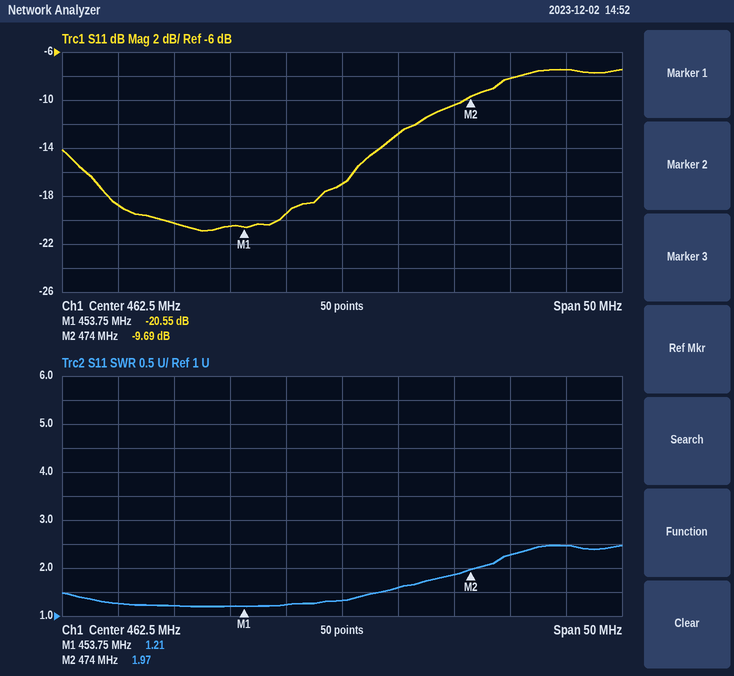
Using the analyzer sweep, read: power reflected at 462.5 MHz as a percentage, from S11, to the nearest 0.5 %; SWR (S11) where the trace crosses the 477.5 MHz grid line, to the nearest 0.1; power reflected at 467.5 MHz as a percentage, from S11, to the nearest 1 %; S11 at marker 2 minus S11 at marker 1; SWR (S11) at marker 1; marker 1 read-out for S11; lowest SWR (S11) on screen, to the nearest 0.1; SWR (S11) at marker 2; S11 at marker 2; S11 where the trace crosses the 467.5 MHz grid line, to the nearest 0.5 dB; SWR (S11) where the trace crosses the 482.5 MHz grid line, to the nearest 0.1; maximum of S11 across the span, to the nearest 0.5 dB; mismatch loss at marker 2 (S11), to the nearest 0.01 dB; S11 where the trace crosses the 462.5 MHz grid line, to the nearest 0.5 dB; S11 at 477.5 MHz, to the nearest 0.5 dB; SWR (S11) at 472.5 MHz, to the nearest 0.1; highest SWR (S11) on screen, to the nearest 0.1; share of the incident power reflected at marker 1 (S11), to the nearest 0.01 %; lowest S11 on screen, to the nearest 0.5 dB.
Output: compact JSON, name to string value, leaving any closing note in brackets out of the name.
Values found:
{"power reflected at 462.5 MHz as a percentage, from S11, to the nearest 0.5 %": "2.0 %", "SWR (S11) where the trace crosses the 477.5 MHz grid line, to the nearest 0.1": "2.3", "power reflected at 467.5 MHz as a percentage, from S11, to the nearest 1 %": "5 %", "S11 at marker 2 minus S11 at marker 1": "10.86 dB", "SWR (S11) at marker 1": "1.21", "marker 1 read-out for S11": "-20.55 dB", "lowest SWR (S11) on screen, to the nearest 0.1": "1.2", "SWR (S11) at marker 2": "1.97", "S11 at marker 2": "-9.69 dB", "S11 where the trace crosses the 467.5 MHz grid line, to the nearest 0.5 dB": "-13.0 dB", "SWR (S11) where the trace crosses the 482.5 MHz grid line, to the nearest 0.1": "2.5", "maximum of S11 across the span, to the nearest 0.5 dB": "-7.5 dB", "mismatch loss at marker 2 (S11), to the nearest 0.01 dB": "0.49 dB", "S11 where the trace crosses the 462.5 MHz grid line, to the nearest 0.5 dB": "-17.0 dB", "S11 at 477.5 MHz, to the nearest 0.5 dB": "-8.0 dB", "SWR (S11) at 472.5 MHz, to the nearest 0.1": "1.9", "highest SWR (S11) on screen, to the nearest 0.1": "2.5", "share of the incident power reflected at marker 1 (S11), to the nearest 0.01 %": "0.88 %", "lowest S11 on screen, to the nearest 0.5 dB": "-21.0 dB"}
